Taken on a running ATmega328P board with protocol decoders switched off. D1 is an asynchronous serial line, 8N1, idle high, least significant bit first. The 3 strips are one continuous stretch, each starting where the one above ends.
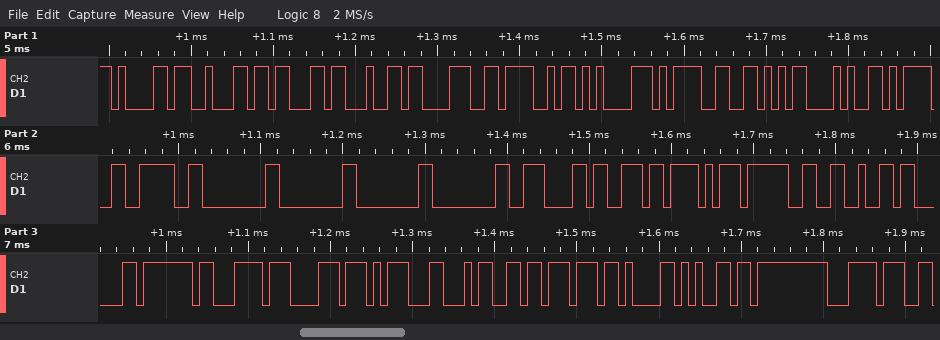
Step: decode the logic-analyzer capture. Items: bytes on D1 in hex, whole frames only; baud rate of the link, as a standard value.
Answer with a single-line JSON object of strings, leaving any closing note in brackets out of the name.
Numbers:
{"bytes on D1 in hex, whole frames only": "0x61 0x62 0x63 0x64 0x38 0x4F 0x85 0x3D 0x56 0x28 0x3D 0x3E 0x00 0x00 0x00 0x00 0x0E 0x73 0xAF 0x3F 0x26 0x03 0x7F 0xBC 0xB8 0x1D 0x34 0xBB 0x0B 0x65 0xFF 0xBC", "baud rate of the link, as a standard value": "115200 baud"}
